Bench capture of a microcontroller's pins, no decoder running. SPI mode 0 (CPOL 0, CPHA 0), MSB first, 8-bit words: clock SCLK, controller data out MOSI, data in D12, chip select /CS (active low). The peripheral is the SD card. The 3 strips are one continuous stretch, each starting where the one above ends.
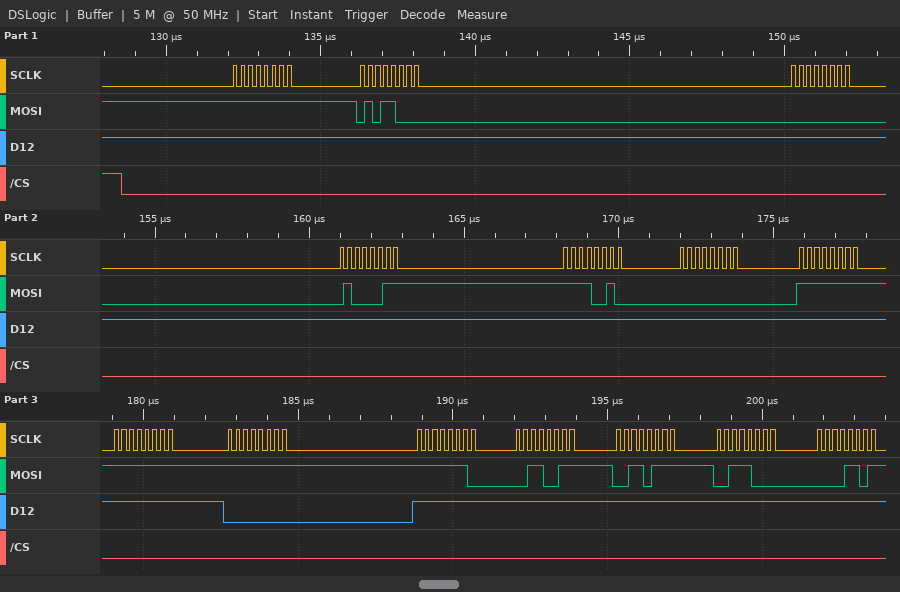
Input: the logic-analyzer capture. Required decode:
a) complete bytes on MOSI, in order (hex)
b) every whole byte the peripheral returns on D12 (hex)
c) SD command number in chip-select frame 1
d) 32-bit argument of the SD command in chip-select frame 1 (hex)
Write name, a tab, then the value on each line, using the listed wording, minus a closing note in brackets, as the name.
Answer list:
complete bytes on MOSI, in order	FF 58 00 43 F2 00 FF FF FF FE 33 37 38 0D
every whole byte the peripheral returns on D12	FF FF FF FF FF FF FF FF 00 FF FF FF FF FF
SD command number in chip-select frame 1	CMD24
32-bit argument of the SD command in chip-select frame 1	0x0043F200
